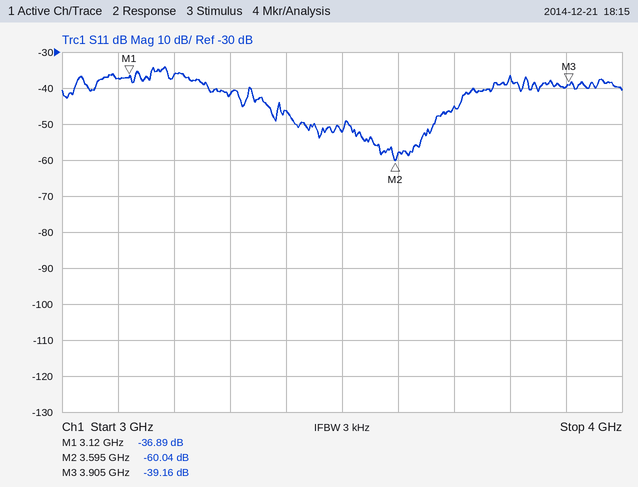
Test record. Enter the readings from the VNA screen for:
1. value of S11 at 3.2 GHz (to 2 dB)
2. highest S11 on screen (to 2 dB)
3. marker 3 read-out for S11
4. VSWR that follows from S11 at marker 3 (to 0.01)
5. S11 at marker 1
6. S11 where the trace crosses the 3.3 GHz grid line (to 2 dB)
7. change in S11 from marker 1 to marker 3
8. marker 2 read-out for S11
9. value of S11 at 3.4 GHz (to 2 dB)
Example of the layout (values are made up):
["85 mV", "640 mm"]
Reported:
["-36 dB", "-34 dB", "-39.16 dB", "1.02", "-36.89 dB", "-42 dB", "-2.27 dB", "-60.04 dB", "-46 dB"]
